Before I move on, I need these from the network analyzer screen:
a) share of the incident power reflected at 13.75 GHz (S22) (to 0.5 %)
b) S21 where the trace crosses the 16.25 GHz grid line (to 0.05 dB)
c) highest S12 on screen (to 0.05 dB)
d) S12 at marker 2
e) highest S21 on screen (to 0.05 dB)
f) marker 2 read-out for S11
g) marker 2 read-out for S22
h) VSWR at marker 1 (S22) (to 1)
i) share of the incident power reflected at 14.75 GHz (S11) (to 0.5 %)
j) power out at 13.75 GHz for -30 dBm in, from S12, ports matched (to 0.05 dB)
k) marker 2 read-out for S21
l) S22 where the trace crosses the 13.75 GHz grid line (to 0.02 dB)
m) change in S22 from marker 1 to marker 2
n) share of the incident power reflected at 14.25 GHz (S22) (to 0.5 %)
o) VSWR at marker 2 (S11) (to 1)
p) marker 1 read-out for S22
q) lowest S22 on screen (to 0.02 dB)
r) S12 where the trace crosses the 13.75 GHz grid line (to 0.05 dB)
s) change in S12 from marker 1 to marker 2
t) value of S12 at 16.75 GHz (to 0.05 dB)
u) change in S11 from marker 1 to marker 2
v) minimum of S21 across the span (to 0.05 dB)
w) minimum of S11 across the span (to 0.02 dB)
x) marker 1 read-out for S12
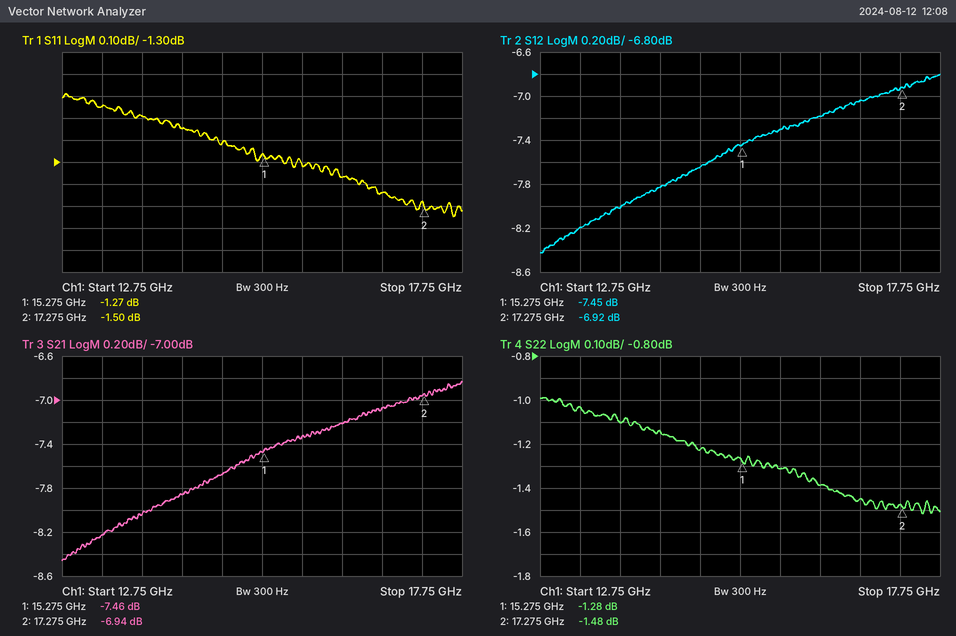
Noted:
77.5 %
-7.20 dB
-6.80 dB
-6.92 dB
-6.85 dB
-1.50 dB
-1.48 dB
14
75.5 %
-38.00 dBm
-6.94 dB
-1.10 dB
-0.20 dB
77.0 %
12
-1.28 dB
-1.52 dB
-8.00 dB
0.53 dB
-7.05 dB
-0.23 dB
-8.45 dB
-1.54 dB
-7.45 dB
